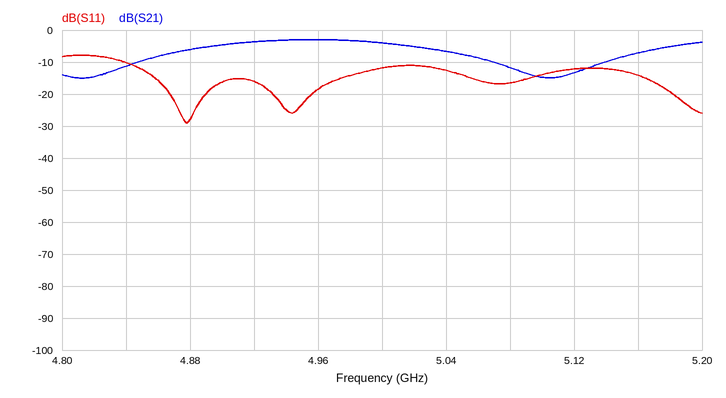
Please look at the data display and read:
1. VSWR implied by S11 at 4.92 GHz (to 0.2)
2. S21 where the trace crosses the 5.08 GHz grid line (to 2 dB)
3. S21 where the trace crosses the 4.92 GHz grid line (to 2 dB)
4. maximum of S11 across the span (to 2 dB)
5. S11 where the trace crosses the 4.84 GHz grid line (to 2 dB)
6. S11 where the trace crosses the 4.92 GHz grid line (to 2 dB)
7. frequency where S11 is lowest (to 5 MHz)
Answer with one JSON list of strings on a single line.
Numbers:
["1.4", "-12 dB", "-4 dB", "-8 dB", "-10 dB", "-16 dB", "4.880 GHz"]
